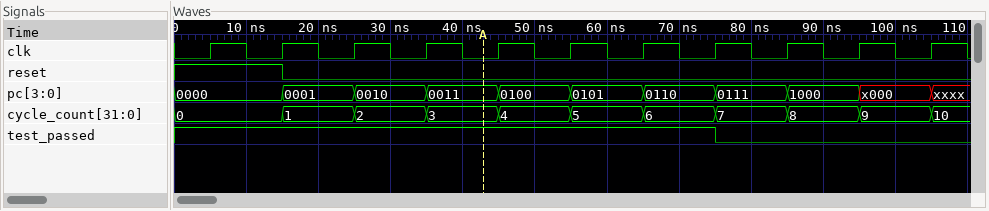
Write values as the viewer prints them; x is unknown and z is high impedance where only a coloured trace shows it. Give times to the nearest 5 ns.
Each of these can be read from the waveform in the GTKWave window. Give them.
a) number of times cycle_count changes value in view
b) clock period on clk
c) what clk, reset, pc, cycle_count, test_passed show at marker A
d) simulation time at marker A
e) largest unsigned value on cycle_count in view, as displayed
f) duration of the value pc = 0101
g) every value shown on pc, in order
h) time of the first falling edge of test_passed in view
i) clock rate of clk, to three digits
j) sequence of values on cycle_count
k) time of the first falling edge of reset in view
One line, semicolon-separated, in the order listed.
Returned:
10; 10 ns; clk=0, reset=0, pc=0011, cycle_count=3, test_passed=1; 45 ns; 10; 10 ns; 0000, 0001, 0010, 0011, 0100, 0101, 0110, 0111, 1000, x000, xxxx; 75 ns; 100 MHz; 0, 1, 2, 3, 4, 5, 6, 7, 8, 9, 10; 15 ns
